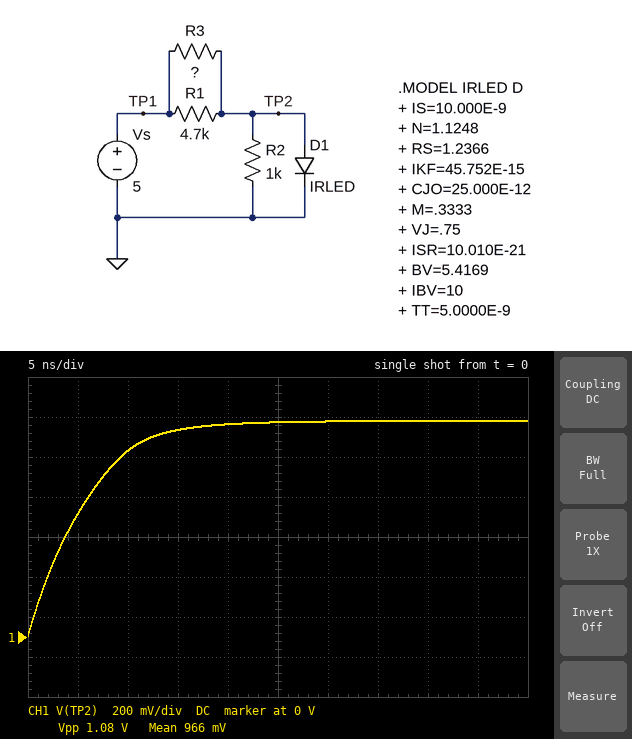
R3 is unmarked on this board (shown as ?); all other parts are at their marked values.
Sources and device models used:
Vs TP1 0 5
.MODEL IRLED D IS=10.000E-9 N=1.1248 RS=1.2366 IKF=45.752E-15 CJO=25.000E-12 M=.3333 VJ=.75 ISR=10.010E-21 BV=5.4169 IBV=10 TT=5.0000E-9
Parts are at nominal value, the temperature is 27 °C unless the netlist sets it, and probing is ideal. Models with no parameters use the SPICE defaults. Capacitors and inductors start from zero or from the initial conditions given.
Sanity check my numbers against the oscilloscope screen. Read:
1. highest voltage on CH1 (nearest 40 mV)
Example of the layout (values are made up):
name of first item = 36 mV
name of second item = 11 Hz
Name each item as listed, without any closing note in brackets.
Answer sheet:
highest voltage on CH1 = 1.08 V
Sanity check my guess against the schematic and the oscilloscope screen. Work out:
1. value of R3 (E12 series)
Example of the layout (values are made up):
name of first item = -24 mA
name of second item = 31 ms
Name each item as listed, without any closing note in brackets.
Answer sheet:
value of R3 = 1.5 kΩ
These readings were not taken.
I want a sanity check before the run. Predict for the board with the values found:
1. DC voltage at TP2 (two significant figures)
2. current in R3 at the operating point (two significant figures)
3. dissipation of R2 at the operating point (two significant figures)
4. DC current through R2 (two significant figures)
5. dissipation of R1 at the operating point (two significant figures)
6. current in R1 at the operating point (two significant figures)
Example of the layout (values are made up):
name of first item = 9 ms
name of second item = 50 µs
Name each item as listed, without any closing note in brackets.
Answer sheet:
DC voltage at TP2 = 1.1 V
current in R3 at the operating point = 2.6 mA
dissipation of R2 at the operating point = 1.2 mW
DC current through R2 = 1.1 mA
dissipation of R1 at the operating point = 3.3 mW
current in R1 at the operating point = 830 µA
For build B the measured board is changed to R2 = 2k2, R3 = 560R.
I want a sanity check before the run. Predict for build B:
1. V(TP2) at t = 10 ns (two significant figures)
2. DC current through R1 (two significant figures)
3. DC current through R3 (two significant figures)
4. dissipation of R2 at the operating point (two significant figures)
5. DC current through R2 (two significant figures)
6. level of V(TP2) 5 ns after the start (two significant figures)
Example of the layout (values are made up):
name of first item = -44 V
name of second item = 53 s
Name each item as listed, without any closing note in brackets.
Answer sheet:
V(TP2) at t = 10 ns = 1.1 V
DC current through R1 = 820 µA
DC current through R3 = 6.9 mA
dissipation of R2 at the operating point = 600 µW
DC current through R2 = 520 µA
level of V(TP2) 5 ns after the start = 1.0 V
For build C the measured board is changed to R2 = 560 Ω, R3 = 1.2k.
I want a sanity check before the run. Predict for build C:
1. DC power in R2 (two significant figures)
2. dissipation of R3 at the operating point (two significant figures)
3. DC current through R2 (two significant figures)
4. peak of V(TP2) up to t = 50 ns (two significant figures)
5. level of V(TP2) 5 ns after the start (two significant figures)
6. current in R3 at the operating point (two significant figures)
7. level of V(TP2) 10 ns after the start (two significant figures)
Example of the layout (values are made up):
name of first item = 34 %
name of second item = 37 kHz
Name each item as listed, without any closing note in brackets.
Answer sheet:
DC power in R2 = 2.1 mW
dissipation of R3 at the operating point = 13 mW
DC current through R2 = 1.9 mA
peak of V(TP2) up to t = 50 ns = 1.1 V
level of V(TP2) 5 ns after the start = 670 mV
current in R3 at the operating point = 3.3 mA
level of V(TP2) 10 ns after the start = 960 mV
